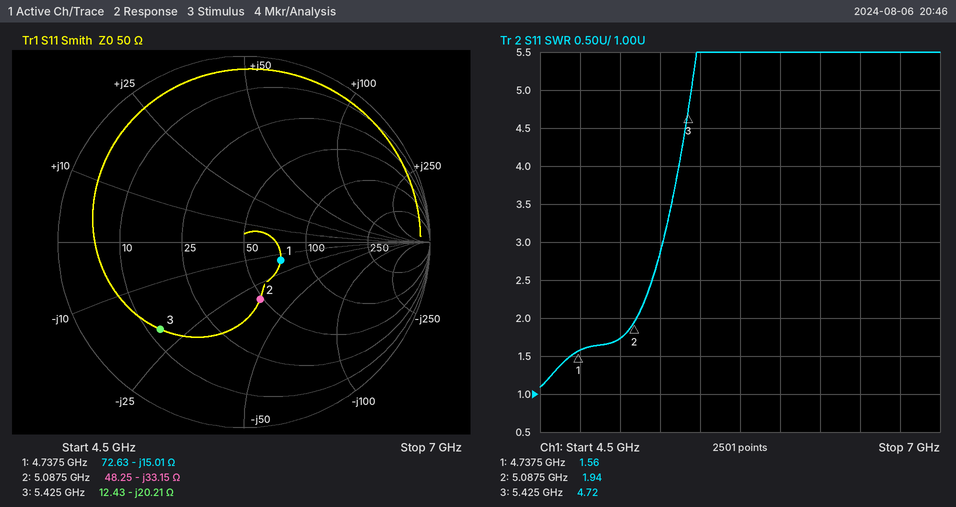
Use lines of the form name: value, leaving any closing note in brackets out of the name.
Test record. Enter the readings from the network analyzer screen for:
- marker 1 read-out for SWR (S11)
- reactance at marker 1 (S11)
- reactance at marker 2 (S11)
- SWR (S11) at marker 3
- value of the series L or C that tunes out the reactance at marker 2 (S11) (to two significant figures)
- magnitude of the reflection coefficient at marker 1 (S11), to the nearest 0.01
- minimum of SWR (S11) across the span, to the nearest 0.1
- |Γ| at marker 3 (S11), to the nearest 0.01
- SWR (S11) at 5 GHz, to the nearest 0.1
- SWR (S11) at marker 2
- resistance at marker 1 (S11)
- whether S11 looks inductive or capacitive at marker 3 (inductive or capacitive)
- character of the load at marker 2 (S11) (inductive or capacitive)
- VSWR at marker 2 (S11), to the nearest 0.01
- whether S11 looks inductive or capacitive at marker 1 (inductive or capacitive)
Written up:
marker 1 read-out for SWR: 1.56
reactance at marker 1: -15.01 Ω
reactance at marker 2: -33.15 Ω
SWR (S11) at marker 3: 4.72
value of the series L or C that tunes out the reactance at marker 2 (S11): 1.0 nH
magnitude of the reflection coefficient at marker 1 (S11), to the nearest 0.01: 0.22
minimum of SWR (S11) across the span, to the nearest 0.1: 1.1
|Γ| at marker 3 (S11), to the nearest 0.01: 0.65
SWR (S11) at 5 GHz, to the nearest 0.1: 1.7
SWR (S11) at marker 2: 1.94
resistance at marker 1: 72.63 Ω
whether S11 looks inductive or capacitive at marker 3: capacitive
character of the load at marker 2 (S11): capacitive
VSWR at marker 2 (S11), to the nearest 0.01: 1.94
whether S11 looks inductive or capacitive at marker 1: capacitive
